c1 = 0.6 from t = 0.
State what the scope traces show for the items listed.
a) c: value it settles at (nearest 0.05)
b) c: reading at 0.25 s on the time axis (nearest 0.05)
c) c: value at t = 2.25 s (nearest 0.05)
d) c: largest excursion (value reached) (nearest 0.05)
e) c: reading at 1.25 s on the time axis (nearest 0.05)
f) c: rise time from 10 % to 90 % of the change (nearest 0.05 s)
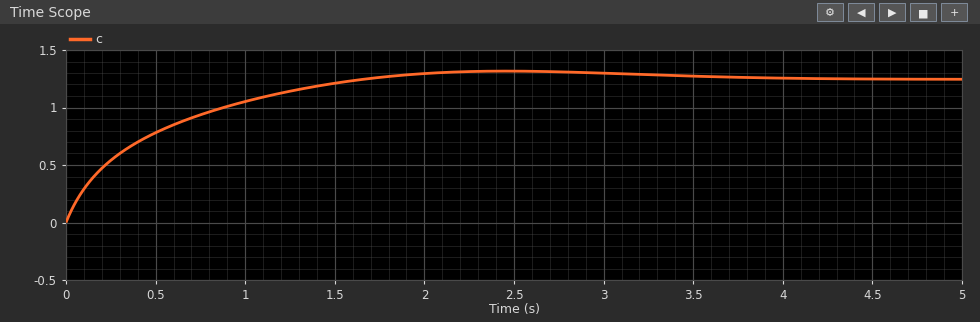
1.25
0.55
1.30
1.30
1.15
1.15 s
